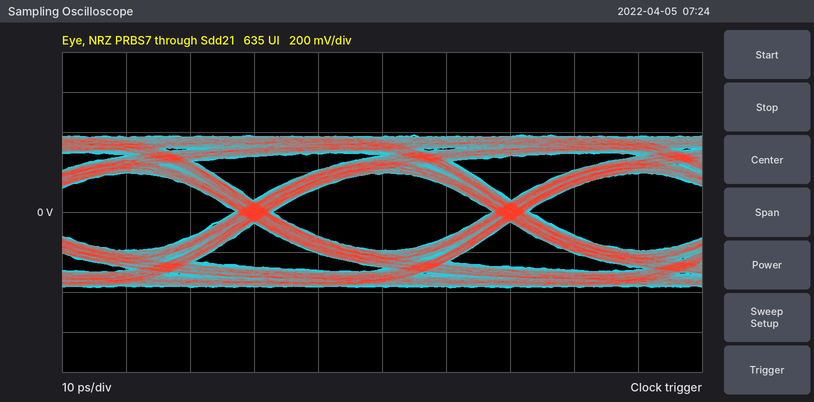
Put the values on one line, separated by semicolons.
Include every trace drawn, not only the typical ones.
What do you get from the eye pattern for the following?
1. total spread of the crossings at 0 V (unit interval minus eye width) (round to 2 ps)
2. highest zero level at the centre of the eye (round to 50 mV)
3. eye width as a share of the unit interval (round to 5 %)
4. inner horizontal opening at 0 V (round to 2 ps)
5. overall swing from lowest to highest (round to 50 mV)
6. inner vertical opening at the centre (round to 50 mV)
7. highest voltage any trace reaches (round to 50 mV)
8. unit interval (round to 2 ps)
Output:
6 ps; -200 mV; 85 %; 34 ps; 750 mV; 400 mV; 400 mV; 40 ps
